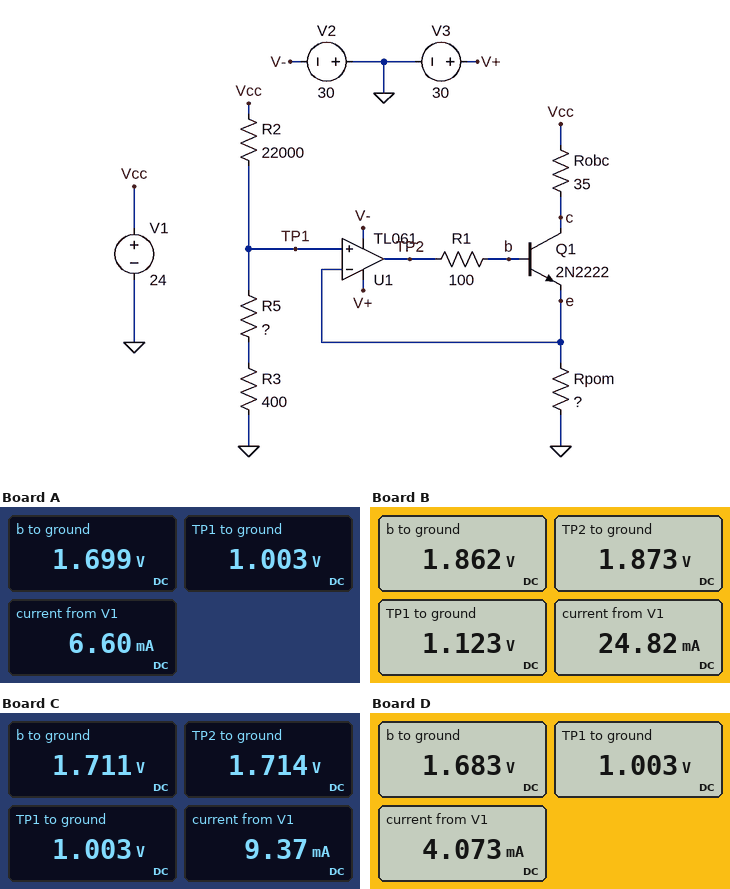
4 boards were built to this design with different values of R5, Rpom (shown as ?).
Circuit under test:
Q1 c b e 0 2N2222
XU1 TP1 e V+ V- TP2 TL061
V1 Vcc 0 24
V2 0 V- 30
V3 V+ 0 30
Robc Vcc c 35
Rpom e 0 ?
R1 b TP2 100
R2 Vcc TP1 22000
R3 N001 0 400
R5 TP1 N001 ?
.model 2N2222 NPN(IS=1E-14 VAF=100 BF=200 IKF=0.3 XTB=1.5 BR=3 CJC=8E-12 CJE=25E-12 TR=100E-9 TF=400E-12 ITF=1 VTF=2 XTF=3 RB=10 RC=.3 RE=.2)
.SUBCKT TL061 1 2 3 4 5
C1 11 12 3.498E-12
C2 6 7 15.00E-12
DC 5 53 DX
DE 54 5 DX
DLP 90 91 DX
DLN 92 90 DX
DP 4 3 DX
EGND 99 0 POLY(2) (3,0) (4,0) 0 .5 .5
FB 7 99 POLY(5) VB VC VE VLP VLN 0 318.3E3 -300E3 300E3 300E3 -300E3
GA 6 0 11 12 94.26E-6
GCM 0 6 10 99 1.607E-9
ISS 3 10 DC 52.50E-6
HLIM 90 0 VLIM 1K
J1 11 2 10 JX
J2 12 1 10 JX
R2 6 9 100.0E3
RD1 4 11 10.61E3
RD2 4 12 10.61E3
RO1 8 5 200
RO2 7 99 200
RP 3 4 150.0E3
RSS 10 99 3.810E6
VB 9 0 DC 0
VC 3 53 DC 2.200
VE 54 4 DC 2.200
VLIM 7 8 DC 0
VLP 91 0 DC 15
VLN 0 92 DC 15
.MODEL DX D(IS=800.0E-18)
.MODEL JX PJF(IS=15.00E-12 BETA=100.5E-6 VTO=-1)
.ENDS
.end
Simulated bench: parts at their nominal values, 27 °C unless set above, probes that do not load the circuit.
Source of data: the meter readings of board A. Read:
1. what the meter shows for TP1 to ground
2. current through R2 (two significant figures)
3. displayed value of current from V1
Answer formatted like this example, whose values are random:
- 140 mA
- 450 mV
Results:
- 1.003 V
- 1.0 mA
- 6.60 mA
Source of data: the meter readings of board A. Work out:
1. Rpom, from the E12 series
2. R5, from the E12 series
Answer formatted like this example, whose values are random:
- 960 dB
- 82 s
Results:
- 180 Ω
- 560 Ω
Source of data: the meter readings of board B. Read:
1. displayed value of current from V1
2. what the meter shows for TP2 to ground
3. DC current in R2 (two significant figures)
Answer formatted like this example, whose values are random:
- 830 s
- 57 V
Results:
- 24.82 mA
- 1.873 V
- 1.0 mA
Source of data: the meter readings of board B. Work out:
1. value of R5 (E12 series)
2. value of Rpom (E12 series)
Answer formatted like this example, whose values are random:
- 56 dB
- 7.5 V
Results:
- 680 Ω
- 47 Ω
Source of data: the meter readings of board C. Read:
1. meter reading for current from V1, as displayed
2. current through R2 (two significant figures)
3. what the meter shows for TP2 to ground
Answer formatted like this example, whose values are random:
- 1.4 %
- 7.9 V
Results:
- 9.37 mA
- 1.0 mA
- 1.714 V
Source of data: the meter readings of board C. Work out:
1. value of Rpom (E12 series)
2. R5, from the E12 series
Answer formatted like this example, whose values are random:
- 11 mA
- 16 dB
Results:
- 120 Ω
- 560 Ω
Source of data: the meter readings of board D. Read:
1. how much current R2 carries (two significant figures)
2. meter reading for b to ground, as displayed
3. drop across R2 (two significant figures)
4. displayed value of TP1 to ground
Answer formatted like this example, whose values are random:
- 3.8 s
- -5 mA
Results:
- 1.0 mA
- 1.683 V
- 23 V
- 1.003 V
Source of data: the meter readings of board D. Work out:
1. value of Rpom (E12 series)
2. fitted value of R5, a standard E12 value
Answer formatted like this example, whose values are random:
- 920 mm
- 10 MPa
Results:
- 330 Ω
- 560 Ω
